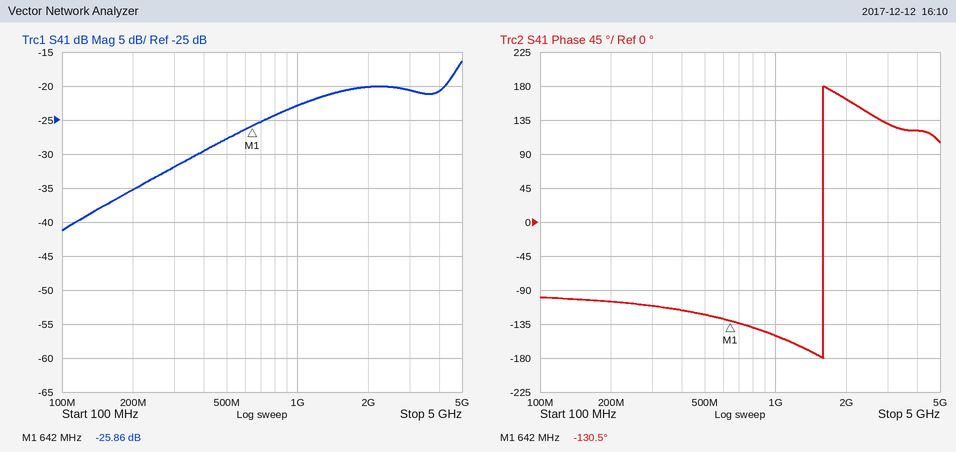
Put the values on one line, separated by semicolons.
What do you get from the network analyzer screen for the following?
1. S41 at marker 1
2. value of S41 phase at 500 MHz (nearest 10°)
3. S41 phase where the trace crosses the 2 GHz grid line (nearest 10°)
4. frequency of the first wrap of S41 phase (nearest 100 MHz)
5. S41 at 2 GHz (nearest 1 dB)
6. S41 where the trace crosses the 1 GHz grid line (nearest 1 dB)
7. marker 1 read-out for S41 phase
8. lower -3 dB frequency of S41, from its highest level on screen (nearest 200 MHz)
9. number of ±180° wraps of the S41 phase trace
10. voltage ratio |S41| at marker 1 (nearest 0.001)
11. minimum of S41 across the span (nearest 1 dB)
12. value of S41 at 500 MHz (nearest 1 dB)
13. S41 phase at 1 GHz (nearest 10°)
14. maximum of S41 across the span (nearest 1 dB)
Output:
-25.86 dB; -120°; 160°; 1.6 GHz; -20 dB; -23 dB; -130.5°; 4.4 GHz; 1; 0.051; -41 dB; -28 dB; -150°; -16 dB
